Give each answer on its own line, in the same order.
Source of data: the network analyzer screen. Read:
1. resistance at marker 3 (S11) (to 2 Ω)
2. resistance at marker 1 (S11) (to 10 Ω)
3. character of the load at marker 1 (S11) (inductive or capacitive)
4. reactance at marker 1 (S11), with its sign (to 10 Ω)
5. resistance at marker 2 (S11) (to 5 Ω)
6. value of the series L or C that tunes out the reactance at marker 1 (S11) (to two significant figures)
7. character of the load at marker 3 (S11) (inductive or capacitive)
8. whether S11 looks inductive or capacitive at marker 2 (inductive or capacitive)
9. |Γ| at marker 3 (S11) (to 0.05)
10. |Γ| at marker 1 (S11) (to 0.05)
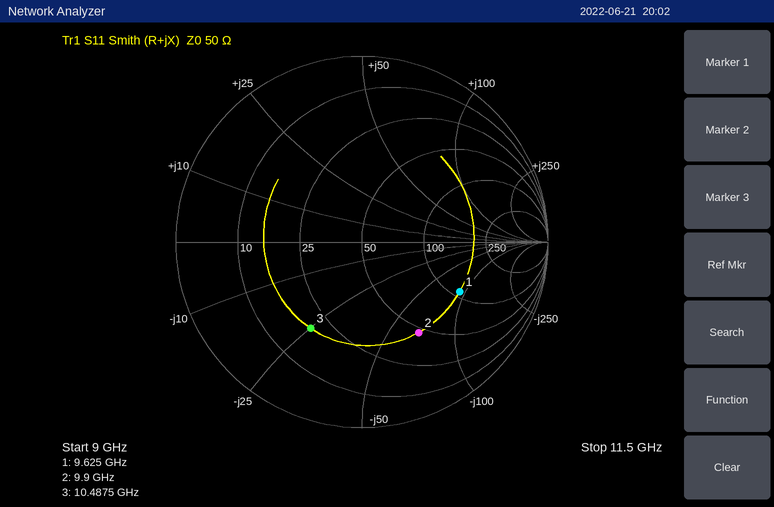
20 Ω
110 Ω
capacitive
-90 Ω
45 Ω
1.5 nH
capacitive
capacitive
0.55
0.60
